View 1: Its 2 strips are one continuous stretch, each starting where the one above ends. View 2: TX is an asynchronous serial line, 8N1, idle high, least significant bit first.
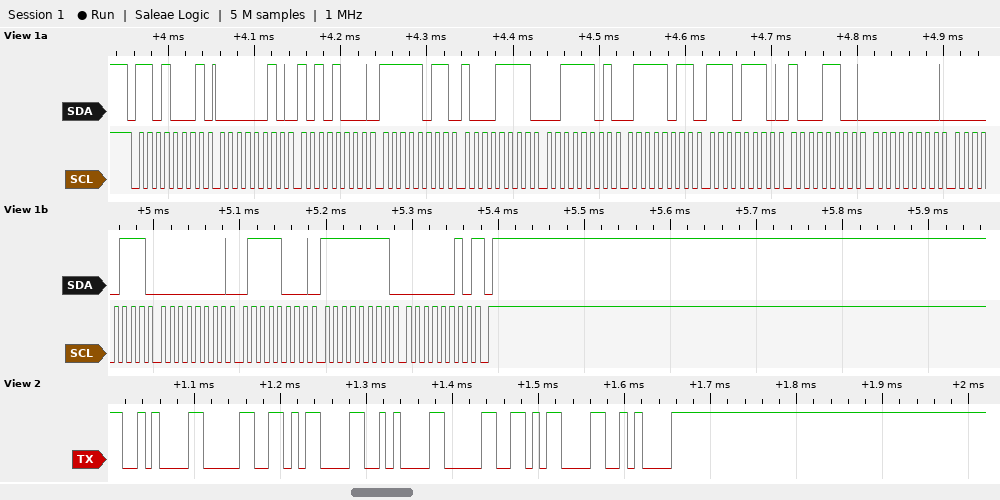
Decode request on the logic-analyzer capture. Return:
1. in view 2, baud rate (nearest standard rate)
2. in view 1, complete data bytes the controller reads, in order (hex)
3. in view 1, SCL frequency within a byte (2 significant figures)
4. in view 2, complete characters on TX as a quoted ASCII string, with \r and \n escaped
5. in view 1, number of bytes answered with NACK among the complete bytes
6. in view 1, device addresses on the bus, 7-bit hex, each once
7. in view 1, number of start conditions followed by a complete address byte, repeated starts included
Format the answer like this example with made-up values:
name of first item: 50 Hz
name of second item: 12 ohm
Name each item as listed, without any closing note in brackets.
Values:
in view 2, baud rate: 115200 baud
in view 1, complete data bytes the controller reads, in order: 02 A8 FB 8F 3D 7B EE 8C 00 07 00 78 FF 02
in view 1, SCL frequency within a byte: 100 kHz
in view 2, complete characters on TX as a quoted ASCII string, with \r and \n escaped: "\n0\r\n0\r\n"
in view 1, number of bytes answered with NACK among the complete bytes: 1
in view 1, device addresses on the bus, 7-bit hex, each once: 0x68
in view 1, number of start conditions followed by a complete address byte, repeated starts included: 1
